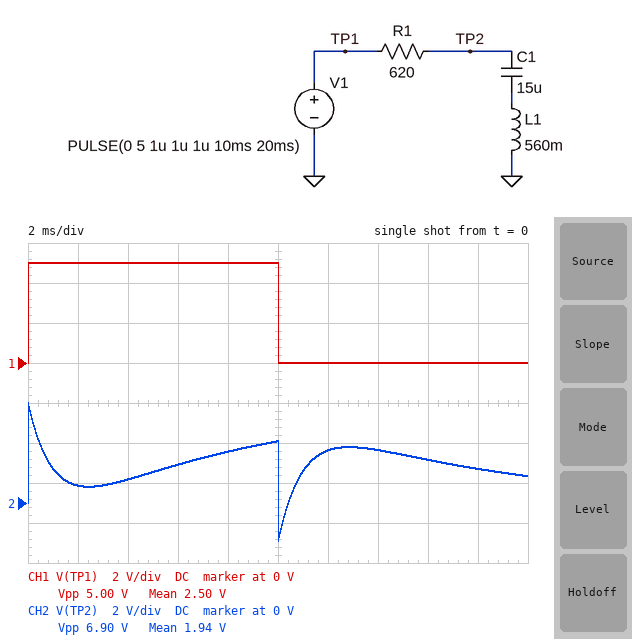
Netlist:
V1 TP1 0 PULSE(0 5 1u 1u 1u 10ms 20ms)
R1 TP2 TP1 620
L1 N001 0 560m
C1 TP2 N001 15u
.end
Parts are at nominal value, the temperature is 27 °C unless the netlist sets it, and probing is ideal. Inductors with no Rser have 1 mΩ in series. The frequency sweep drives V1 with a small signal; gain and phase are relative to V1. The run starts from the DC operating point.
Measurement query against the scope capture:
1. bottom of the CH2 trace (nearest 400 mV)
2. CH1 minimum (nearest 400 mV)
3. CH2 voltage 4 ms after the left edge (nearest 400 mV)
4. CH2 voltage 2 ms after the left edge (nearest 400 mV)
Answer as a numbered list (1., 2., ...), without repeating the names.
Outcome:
1. -2.0 V
2. 0 V
3. 1.2 V
4. 800 mV
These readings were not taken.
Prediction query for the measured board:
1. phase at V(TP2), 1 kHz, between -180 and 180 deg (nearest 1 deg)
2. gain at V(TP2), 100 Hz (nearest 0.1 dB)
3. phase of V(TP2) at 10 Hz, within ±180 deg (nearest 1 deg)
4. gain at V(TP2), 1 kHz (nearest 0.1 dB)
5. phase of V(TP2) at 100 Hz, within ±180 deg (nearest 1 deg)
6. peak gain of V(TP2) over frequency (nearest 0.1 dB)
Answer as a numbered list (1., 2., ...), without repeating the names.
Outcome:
1. 10 deg
2. -8.7 dB
3. -31 deg
4. -0.1 dB
5. 68 deg
6. 0 dB
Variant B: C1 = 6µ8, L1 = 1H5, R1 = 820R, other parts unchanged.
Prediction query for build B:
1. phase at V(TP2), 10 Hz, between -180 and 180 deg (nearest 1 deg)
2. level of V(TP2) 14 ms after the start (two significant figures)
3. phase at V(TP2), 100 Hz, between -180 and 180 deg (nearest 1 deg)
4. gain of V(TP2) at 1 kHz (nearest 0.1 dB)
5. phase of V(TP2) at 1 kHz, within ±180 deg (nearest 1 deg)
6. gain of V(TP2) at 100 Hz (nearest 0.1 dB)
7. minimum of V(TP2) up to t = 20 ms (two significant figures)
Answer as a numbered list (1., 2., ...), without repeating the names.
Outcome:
1. -20 deg
2. 3.1 V
3. 49 deg
4. 0 dB
5. 5 deg
6. -3.7 dB
7. -1.2 V
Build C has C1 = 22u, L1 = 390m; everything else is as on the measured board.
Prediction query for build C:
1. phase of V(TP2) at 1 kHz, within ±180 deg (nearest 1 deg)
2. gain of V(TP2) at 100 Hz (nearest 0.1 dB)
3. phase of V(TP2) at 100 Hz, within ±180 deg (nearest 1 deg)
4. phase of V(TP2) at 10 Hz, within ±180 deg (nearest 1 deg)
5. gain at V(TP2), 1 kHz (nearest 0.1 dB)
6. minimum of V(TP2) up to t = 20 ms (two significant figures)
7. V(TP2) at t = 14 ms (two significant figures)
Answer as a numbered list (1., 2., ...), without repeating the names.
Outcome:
1. 14 deg
2. -11.4 dB
3. 74 deg
4. -42 deg
5. -0.3 dB
6. -2.6 V
7. 2.2 V
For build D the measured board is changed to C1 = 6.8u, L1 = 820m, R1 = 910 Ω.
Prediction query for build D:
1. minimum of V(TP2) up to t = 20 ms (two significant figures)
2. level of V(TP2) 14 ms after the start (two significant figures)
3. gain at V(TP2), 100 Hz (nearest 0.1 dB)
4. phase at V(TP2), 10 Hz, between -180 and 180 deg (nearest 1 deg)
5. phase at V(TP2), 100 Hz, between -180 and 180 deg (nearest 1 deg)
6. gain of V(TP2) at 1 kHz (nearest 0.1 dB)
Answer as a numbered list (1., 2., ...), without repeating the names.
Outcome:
1. -1.1 V
2. 2.8 V
3. -10.6 dB
4. -22 deg
5. 73 deg
6. -0.1 dB
